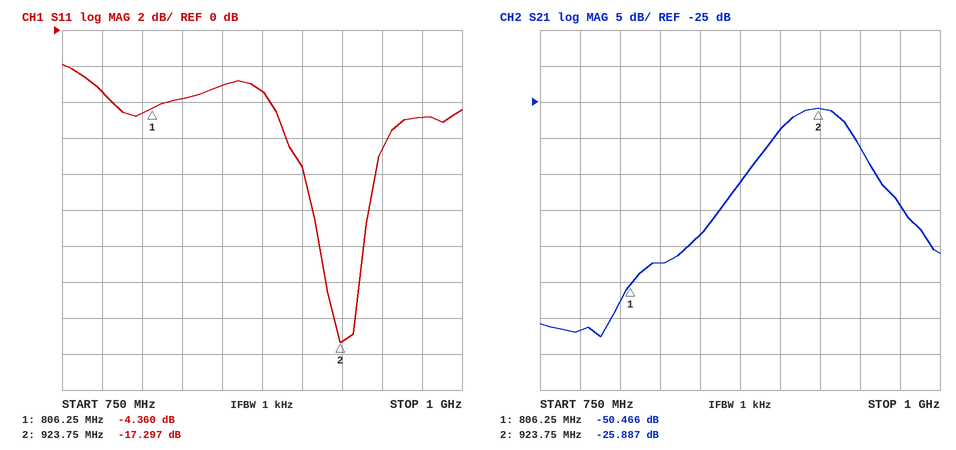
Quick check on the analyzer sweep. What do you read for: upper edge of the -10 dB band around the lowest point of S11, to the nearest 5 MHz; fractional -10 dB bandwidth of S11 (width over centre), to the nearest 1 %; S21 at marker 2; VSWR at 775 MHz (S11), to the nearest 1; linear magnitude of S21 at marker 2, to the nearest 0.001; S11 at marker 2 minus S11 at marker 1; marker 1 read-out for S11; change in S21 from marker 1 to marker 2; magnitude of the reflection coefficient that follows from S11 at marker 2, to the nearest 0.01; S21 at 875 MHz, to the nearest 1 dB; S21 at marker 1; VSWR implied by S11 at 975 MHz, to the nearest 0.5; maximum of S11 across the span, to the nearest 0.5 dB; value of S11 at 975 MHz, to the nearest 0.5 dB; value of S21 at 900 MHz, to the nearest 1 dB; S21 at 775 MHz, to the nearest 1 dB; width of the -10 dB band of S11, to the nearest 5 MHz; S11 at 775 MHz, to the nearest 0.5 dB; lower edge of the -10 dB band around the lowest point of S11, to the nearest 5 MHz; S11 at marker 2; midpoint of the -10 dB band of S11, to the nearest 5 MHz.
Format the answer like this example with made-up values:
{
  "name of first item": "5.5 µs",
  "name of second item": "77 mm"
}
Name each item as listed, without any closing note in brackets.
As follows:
{
  "upper edge of the -10 dB band around the lowest point of S11, to the nearest 5 MHz": "940 MHz",
  "fractional -10 dB bandwidth of S11 (width over centre), to the nearest 1 %": "4 %",
  "S21 at marker 2": "-25.887 dB",
  "VSWR at 775 MHz (S11), to the nearest 1": "5",
  "linear magnitude of S21 at marker 2, to the nearest 0.001": "0.051",
  "S11 at marker 2 minus S11 at marker 1": "-12.937 dB",
  "marker 1 read-out for S11": "-4.360 dB",
  "change in S21 from marker 1 to marker 2": "24.579 dB",
  "magnitude of the reflection coefficient that follows from S11 at marker 2, to the nearest 0.01": "0.14",
  "S21 at 875 MHz, to the nearest 1 dB": "-36 dB",
  "S21 at marker 1": "-50.466 dB",
  "VSWR implied by S11 at 975 MHz, to the nearest 0.5": "3.5",
  "maximum of S11 across the span, to the nearest 0.5 dB": "-2.0 dB",
  "value of S11 at 975 MHz, to the nearest 0.5 dB": "-5.0 dB",
  "value of S21 at 900 MHz, to the nearest 1 dB": "-29 dB",
  "S21 at 775 MHz, to the nearest 1 dB": "-57 dB",
  "width of the -10 dB band of S11, to the nearest 5 MHz": "35 MHz",
  "S11 at 775 MHz, to the nearest 0.5 dB": "-3.5 dB",
  "lower edge of the -10 dB band around the lowest point of S11, to the nearest 5 MHz": "905 MHz",
  "S11 at marker 2": "-17.297 dB",
  "midpoint of the -10 dB band of S11, to the nearest 5 MHz": "925 MHz"
}
